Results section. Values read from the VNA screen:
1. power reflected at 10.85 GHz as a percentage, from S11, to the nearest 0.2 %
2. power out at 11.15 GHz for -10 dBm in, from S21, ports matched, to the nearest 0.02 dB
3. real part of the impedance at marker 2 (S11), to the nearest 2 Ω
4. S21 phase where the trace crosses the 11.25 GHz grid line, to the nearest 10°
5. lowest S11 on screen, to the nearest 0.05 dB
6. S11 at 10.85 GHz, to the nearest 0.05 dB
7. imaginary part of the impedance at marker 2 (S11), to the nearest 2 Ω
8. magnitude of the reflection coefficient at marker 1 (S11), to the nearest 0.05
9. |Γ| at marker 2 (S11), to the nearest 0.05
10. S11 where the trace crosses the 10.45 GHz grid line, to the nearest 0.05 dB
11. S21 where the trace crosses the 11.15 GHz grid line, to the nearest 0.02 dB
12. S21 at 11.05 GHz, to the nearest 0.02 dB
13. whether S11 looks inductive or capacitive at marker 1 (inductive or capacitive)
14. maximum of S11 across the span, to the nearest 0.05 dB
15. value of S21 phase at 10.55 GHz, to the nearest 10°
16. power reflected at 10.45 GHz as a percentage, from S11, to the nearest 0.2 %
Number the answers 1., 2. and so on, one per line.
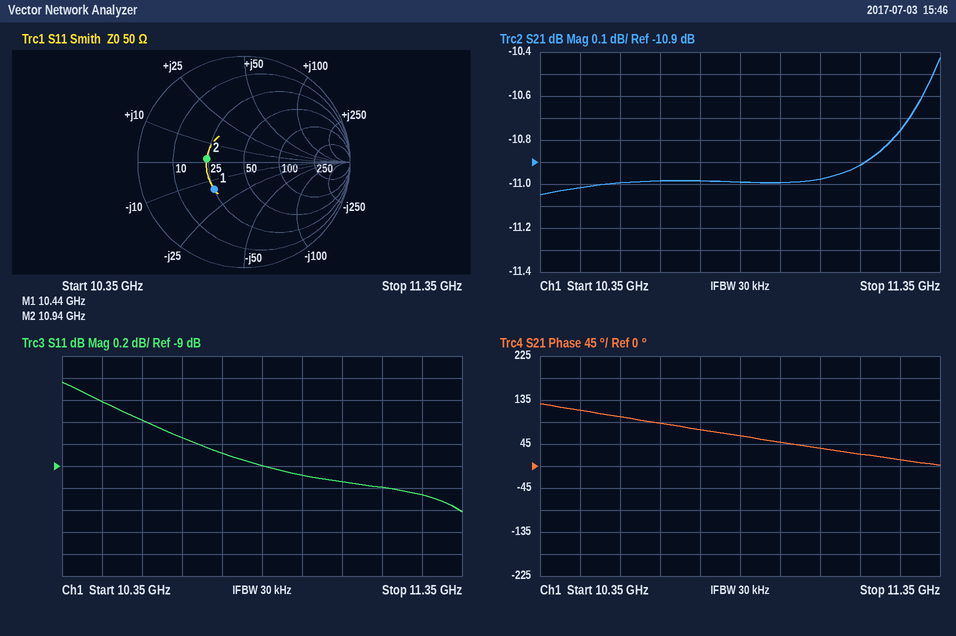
1. 12.6 %
2. -20.92 dBm
3. 24 Ω
4. 10°
5. -9.40 dB
6. -9.00 dB
7. +2 Ω
8. 0.40
9. 0.35
10. -8.40 dB
11. -10.92 dB
12. -10.98 dB
13. capacitive
14. -8.25 dB
15. 100°
16. 14.4 %
